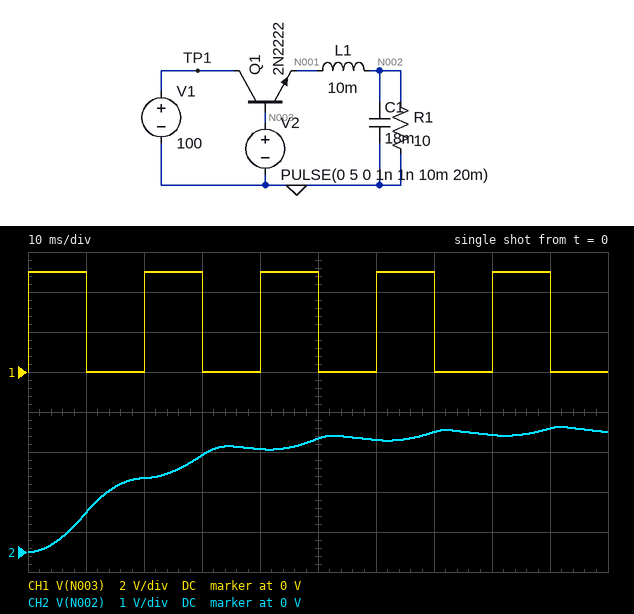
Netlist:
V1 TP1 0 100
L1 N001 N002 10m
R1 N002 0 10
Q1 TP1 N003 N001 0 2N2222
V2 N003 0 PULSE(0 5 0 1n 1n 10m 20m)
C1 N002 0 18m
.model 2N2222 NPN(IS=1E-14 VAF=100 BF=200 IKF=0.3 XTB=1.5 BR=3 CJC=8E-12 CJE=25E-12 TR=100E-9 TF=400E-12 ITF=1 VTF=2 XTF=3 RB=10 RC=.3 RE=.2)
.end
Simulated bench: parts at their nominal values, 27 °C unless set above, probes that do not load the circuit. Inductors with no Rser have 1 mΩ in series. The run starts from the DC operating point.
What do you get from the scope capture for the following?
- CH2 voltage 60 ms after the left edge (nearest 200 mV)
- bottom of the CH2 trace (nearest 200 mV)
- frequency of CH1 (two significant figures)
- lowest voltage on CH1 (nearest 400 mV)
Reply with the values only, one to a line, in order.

2.8 V
0 V
50 Hz
0 V
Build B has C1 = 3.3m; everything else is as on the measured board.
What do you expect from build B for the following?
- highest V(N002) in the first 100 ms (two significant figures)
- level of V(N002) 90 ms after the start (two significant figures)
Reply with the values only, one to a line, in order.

4.8 V
3.7 V
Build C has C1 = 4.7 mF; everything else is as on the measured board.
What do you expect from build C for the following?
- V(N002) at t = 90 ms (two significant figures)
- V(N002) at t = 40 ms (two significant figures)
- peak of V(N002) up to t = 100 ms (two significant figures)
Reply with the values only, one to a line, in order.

3.5 V
3.0 V
4.1 V
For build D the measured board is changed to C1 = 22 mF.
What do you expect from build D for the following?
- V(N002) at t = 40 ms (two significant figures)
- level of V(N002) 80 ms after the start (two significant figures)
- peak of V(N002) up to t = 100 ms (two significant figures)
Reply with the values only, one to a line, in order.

2.4 V
2.8 V
3.0 V
